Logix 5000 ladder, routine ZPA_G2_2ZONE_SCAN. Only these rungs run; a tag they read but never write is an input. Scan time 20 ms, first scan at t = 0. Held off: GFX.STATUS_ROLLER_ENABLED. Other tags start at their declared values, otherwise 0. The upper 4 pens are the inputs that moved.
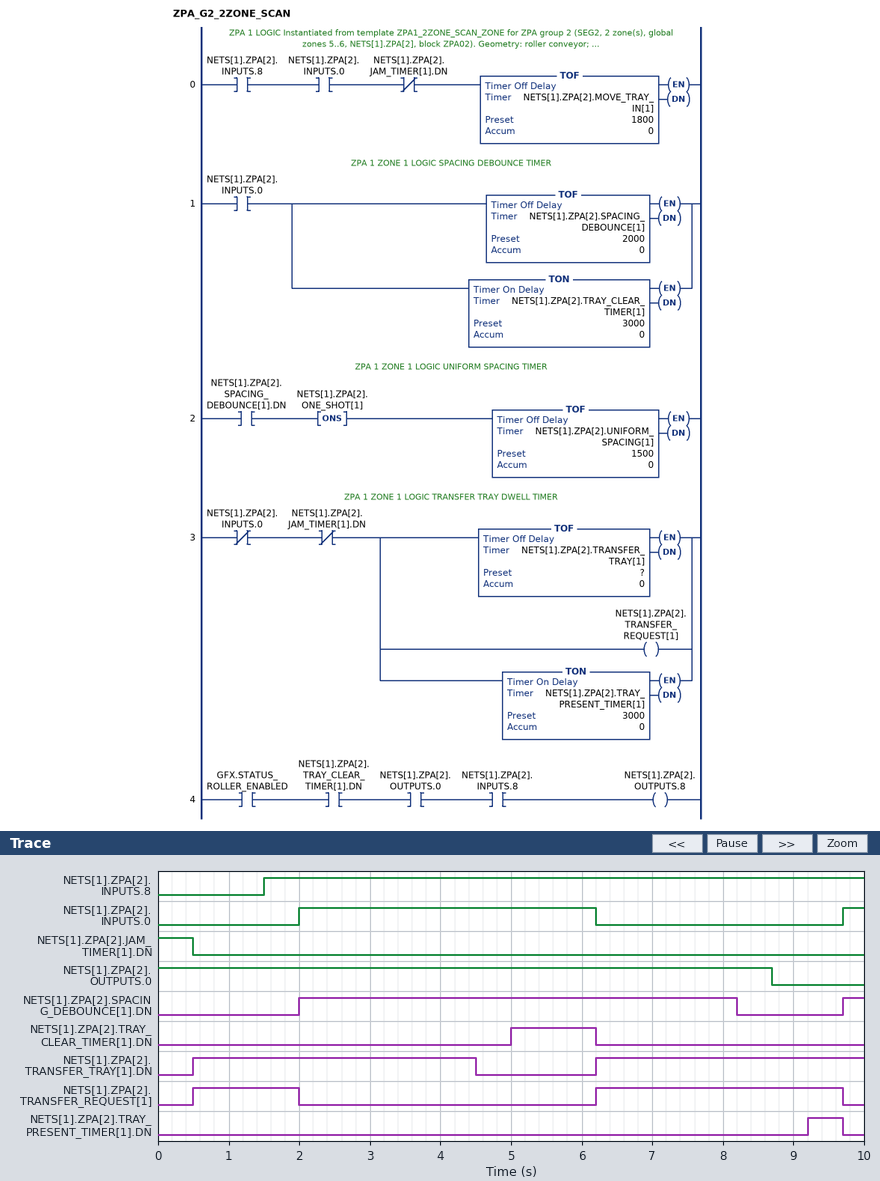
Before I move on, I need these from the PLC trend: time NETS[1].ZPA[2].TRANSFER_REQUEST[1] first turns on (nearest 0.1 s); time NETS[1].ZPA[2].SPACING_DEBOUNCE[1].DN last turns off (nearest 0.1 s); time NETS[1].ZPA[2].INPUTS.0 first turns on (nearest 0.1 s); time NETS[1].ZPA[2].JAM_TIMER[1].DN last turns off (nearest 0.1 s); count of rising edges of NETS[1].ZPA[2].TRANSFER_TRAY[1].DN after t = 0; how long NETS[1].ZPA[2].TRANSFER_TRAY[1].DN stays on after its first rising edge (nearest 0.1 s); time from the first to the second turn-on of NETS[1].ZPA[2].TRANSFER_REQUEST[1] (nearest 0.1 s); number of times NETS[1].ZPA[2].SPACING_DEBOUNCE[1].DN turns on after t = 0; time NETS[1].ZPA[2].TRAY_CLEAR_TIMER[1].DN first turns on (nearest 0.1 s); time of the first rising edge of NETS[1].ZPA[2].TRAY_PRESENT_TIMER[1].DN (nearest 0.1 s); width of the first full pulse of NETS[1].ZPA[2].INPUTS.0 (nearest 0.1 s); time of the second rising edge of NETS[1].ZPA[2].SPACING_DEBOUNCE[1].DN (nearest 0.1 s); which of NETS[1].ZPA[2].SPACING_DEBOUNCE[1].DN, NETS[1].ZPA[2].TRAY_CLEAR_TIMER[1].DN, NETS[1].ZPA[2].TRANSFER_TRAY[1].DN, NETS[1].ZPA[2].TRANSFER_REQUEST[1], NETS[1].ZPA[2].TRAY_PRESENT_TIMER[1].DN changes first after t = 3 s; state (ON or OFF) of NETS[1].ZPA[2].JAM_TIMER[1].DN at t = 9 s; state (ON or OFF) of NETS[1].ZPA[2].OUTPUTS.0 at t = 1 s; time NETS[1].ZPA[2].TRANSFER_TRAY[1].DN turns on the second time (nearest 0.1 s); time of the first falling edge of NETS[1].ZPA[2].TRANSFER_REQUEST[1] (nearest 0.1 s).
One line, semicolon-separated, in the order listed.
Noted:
0.5 s; 8.2 s; 2.0 s; 0.5 s; 2; 4.0 s; 5.7 s; 2; 5.0 s; 9.2 s; 4.2 s; 9.7 s; NETS[1].ZPA[2].TRANSFER_TRAY[1].DN; OFF; ON; 6.2 s; 2.0 s
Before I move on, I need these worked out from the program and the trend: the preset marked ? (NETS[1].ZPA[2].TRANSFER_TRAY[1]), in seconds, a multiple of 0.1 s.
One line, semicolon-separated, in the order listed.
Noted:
2.5 s
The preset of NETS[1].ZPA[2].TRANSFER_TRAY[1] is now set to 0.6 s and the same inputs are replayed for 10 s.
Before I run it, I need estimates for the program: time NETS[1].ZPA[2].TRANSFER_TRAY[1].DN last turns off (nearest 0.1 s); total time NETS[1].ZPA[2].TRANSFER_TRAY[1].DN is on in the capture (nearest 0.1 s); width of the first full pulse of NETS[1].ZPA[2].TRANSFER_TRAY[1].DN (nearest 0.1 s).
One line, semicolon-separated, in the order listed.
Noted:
2.6 s; 5.9 s; 2.1 s
